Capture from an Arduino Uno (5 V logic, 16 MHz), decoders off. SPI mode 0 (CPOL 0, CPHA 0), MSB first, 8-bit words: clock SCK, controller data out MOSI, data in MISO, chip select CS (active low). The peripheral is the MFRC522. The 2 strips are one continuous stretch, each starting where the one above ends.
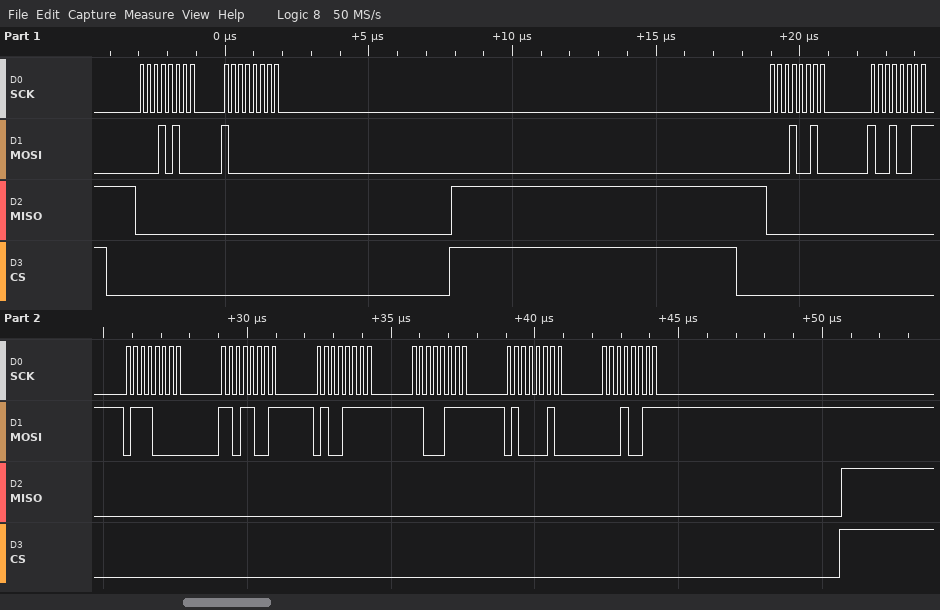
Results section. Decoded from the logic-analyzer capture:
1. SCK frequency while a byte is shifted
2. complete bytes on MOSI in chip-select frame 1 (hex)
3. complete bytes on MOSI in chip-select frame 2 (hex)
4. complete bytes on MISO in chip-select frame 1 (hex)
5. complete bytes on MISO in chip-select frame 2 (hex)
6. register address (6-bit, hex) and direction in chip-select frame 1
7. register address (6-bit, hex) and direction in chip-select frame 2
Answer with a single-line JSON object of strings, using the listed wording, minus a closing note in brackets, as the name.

{"SCK frequency while a byte is shifted": "4 MHz", "complete bytes on MOSI in chip-select frame 1": "0x14 0x80", "complete bytes on MOSI in chip-select frame 2": "0x12 0x93 0x70 0xD9 0x4F 0xC7 0x42 0x13", "complete bytes on MISO in chip-select frame 1": "0x00 0x00", "complete bytes on MISO in chip-select frame 2": "0x00 0x00 0x00 0x00 0x00 0x00 0x00 0x00", "register address (6-bit, hex) and direction in chip-select frame 1": "0x0A write", "register address (6-bit, hex) and direction in chip-select frame 2": "0x09 write"}
